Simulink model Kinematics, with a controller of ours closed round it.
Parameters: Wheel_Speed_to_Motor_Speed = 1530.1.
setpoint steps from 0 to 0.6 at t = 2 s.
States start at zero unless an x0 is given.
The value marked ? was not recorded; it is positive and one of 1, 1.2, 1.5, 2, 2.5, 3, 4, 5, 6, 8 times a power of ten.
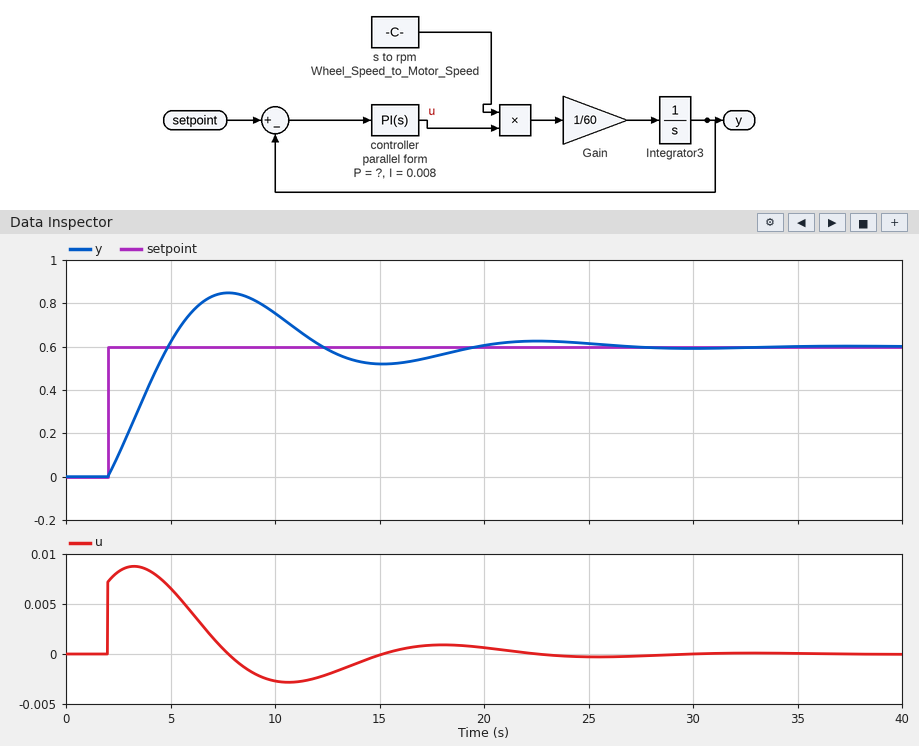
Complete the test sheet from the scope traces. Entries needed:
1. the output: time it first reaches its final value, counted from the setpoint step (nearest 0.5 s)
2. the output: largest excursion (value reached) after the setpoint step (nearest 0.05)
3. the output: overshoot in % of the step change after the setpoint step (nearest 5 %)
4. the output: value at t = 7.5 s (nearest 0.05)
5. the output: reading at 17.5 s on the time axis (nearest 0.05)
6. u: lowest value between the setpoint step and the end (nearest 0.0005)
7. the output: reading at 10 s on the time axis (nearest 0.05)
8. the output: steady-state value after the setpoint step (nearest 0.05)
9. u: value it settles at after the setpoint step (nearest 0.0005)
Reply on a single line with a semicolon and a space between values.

3.0 s; 0.85; 40 %; 0.85; 0.55; -0.0030; 0.75; 0.60; 0.0000
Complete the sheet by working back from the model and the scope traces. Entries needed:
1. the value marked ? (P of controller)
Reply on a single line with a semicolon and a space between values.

0.012
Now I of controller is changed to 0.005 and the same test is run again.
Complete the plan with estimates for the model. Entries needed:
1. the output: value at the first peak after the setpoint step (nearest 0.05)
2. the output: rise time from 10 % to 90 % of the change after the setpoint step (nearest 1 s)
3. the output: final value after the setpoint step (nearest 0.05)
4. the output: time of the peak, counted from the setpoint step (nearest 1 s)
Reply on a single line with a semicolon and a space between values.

0.80; 3 s; 0.60; 7 s
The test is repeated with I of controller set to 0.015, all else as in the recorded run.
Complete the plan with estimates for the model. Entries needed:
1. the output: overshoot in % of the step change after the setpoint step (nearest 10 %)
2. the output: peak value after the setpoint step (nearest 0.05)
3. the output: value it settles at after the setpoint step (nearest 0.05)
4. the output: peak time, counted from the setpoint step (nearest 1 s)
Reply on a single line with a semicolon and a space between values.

50 %; 0.90; 0.60; 4 s
